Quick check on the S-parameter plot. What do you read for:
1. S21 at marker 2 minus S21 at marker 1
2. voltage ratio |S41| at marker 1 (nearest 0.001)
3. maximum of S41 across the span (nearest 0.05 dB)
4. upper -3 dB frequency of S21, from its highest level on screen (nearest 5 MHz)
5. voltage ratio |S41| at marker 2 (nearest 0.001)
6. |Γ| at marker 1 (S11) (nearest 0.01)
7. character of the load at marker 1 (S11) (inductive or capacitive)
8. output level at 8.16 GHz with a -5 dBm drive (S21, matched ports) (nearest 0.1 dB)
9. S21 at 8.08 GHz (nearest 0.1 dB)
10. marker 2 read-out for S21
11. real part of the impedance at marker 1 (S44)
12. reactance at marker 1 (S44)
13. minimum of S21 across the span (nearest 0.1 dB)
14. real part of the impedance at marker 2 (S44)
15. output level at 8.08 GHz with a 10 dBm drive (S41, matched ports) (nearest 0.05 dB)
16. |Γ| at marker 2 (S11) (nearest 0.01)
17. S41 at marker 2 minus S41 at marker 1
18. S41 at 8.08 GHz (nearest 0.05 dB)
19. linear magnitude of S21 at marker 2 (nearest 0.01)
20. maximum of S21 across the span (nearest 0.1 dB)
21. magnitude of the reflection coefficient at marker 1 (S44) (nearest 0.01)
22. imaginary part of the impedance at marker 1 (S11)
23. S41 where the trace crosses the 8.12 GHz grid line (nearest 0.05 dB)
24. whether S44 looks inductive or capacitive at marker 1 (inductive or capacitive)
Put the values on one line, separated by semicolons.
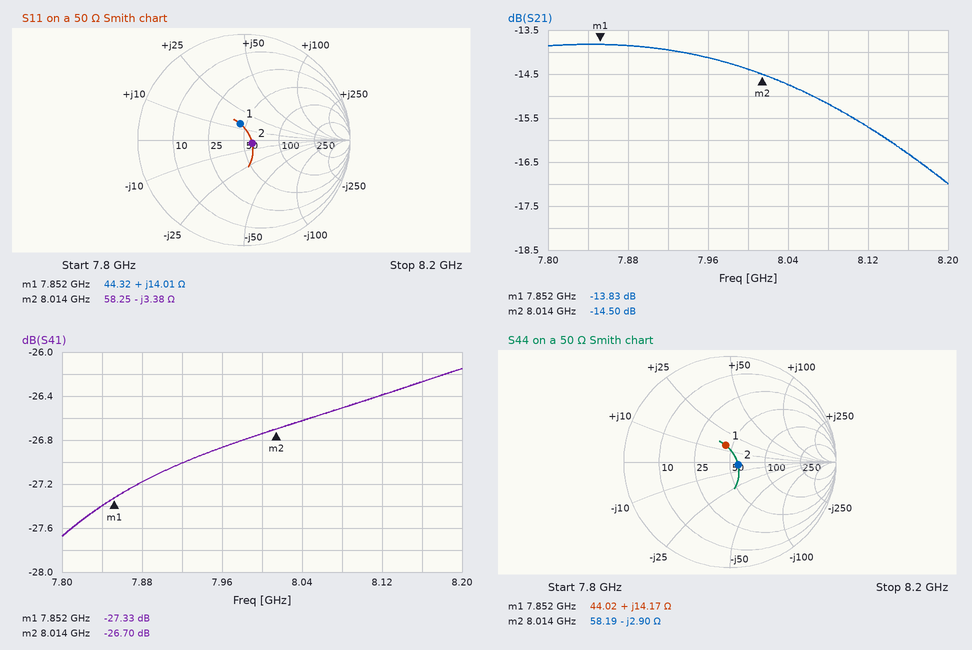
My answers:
-0.67 dB; 0.043; -26.15 dB; 8.190 GHz; 0.046; 0.16; inductive; -21.3 dBm; -15.2 dB; -14.50 dB; 44.02 Ω; +14.17 Ω; -17.0 dB; 58.19 Ω; -16.50 dBm; 0.08; 0.63 dB; -26.50 dB; 0.19; -13.8 dB; 0.16; +14.01 Ω; -26.40 dB; inductive
